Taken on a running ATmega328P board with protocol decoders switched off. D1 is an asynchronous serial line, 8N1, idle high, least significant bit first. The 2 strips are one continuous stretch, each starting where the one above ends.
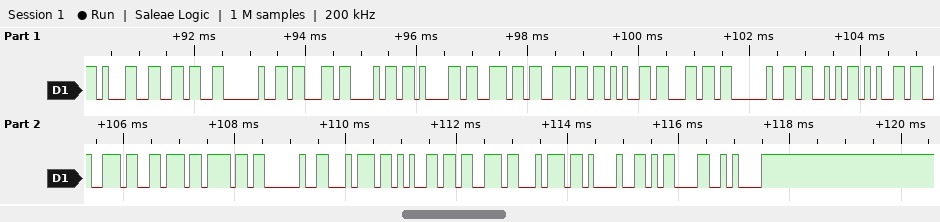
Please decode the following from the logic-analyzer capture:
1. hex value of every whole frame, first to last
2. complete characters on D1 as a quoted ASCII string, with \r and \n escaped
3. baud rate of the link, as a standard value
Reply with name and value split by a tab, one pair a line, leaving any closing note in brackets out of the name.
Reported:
hex value of every whole frame, first to last	0x31 0x36 0x20 0x63 0x68 0x61 0x6E 0x6E 0x65 0x6C 0x20 0x53 0x65 0x72 0x76 0x6F 0x20 0x74 0x65 0x73 0x74 0x21 0x0D 0x0A
complete characters on D1 as a quoted ASCII string, with \r and \n escaped	"16 channel Servo test!\r\n"
baud rate of the link, as a standard value	9600 baud
